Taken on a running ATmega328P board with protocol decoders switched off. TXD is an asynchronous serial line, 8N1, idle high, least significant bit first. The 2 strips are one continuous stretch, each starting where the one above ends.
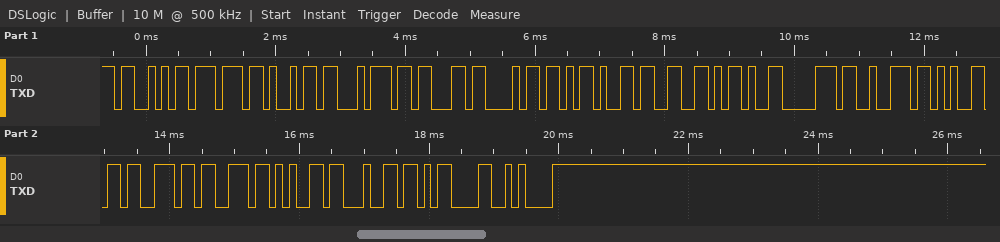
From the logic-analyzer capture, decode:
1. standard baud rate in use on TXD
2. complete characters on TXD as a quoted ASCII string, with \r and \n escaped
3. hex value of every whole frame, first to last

9600 baud
"Switch-3-pressed\r\n"
53 77 69 74 63 68 2D 33 2D 70 72 65 73 73 65 64 0D 0A
